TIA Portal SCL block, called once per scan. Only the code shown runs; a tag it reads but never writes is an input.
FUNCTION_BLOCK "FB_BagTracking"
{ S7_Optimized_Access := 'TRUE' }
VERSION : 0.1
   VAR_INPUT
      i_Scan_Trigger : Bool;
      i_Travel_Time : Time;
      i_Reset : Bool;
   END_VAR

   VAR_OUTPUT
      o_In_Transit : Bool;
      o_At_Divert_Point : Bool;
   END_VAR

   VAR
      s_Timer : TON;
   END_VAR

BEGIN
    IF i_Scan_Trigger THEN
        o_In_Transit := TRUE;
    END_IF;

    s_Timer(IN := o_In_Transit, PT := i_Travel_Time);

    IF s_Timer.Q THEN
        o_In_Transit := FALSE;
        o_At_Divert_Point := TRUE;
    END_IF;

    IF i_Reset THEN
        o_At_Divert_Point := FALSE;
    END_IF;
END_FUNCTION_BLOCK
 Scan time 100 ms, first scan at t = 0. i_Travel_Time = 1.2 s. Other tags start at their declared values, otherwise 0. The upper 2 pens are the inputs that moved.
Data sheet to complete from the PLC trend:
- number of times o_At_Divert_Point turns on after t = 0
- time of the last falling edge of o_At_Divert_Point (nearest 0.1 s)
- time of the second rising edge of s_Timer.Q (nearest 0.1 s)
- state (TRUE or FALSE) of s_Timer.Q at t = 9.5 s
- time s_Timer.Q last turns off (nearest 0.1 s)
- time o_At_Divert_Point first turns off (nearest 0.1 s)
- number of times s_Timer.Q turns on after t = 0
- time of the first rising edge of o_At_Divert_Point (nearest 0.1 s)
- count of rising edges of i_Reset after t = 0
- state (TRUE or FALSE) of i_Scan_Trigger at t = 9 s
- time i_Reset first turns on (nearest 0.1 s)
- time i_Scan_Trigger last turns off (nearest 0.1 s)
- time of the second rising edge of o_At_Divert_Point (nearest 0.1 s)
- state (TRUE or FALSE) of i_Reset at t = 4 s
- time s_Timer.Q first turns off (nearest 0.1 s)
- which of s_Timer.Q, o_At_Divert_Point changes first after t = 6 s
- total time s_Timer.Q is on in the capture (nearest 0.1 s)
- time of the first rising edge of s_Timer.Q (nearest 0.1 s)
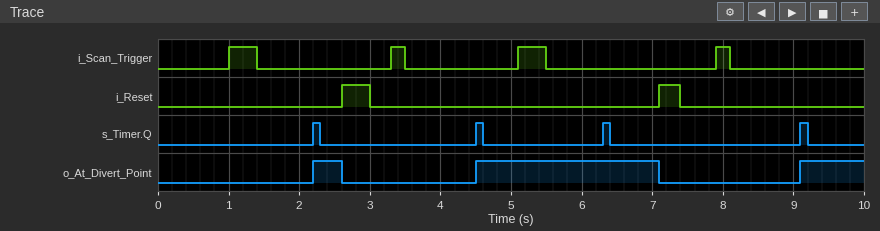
3
7.1 s
4.5 s
FALSE
9.2 s
2.6 s
4
2.2 s
2
FALSE
2.6 s
8.1 s
4.5 s
FALSE
2.3 s
s_Timer.Q
0.4 s
2.2 s
